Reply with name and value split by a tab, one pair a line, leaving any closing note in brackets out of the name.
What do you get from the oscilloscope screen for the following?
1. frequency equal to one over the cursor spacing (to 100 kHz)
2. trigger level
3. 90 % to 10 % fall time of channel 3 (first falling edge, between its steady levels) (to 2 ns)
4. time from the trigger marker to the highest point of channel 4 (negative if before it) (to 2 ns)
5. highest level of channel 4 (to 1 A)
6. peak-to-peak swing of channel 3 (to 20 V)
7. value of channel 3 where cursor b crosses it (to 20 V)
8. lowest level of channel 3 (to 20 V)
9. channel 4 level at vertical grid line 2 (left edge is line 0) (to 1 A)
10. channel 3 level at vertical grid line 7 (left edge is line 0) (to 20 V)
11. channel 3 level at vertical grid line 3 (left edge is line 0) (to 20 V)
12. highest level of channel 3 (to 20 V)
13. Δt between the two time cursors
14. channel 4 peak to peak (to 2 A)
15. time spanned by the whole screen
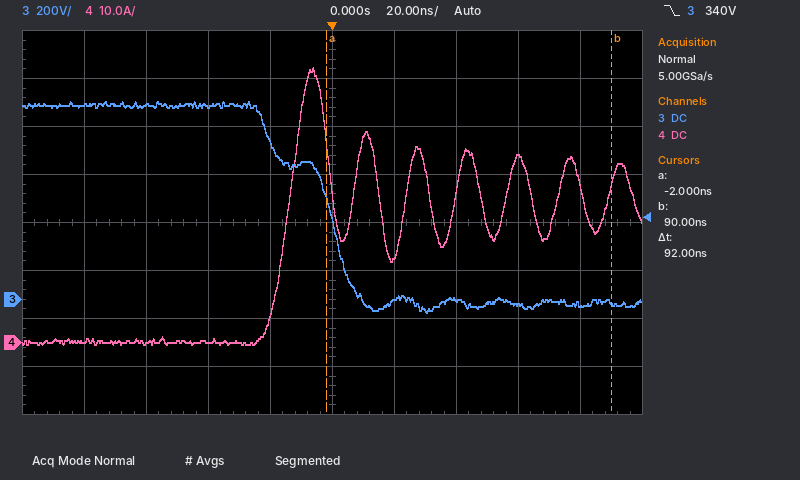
frequency equal to one over the cursor spacing	10.9 MHz
trigger level	340 V
90 % to 10 % fall time of channel 3 (first falling edge, between its steady levels)	28 ns
time from the trigger marker to the highest point of channel 4 (negative if before it)	-6 ns
highest level of channel 4	57 A
peak-to-peak swing of channel 3	880 V
value of channel 3 where cursor b crosses it	-20 V
lowest level of channel 3	-60 V
channel 4 level at vertical grid line 2 (left edge is line 0)	0 A
channel 3 level at vertical grid line 7 (left edge is line 0)	0 V
channel 3 level at vertical grid line 3 (left edge is line 0)	800 V
highest level of channel 3	820 V
Δt between the two time cursors	92 ns
channel 4 peak to peak	58 A
time spanned by the whole screen	200 ns
